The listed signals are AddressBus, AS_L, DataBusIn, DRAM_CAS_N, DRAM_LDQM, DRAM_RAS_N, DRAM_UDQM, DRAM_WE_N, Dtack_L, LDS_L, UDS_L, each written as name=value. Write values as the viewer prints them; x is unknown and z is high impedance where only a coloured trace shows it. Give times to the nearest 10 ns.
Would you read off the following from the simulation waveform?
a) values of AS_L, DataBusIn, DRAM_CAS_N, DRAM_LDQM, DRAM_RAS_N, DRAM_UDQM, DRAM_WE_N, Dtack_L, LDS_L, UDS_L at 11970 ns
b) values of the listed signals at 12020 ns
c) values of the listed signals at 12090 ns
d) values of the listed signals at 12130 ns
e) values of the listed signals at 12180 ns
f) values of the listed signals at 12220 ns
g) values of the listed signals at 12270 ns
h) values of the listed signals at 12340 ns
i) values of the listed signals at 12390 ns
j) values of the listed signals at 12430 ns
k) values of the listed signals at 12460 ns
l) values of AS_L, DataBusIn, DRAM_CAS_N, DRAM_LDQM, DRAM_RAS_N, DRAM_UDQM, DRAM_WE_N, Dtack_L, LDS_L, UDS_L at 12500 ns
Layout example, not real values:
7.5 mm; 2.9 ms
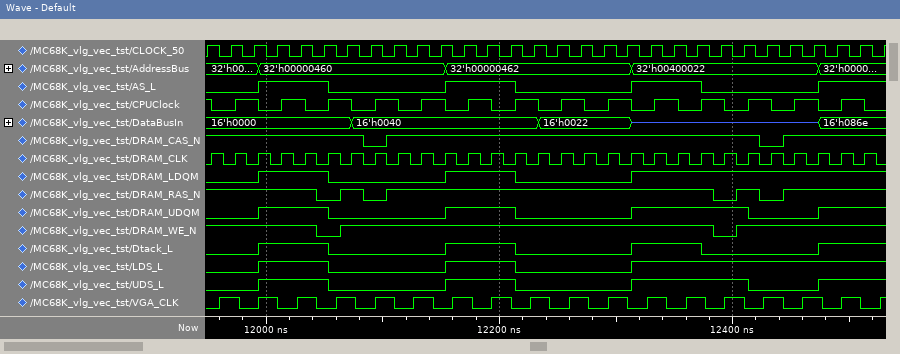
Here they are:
AS_L=0, DataBusIn=16'h0000, DRAM_CAS_N=1, DRAM_LDQM=0, DRAM_RAS_N=1, DRAM_UDQM=0, DRAM_WE_N=1, Dtack_L=0, LDS_L=0, UDS_L=0; AddressBus=32'h00000460, AS_L=1, DataBusIn=16'h0000, DRAM_CAS_N=1, DRAM_LDQM=1, DRAM_RAS_N=1, DRAM_UDQM=1, DRAM_WE_N=1, Dtack_L=1, LDS_L=1, UDS_L=1; AddressBus=32'h00000460, AS_L=0, DataBusIn=16'h0040, DRAM_CAS_N=0, DRAM_LDQM=0, DRAM_RAS_N=0, DRAM_UDQM=0, DRAM_WE_N=1, Dtack_L=0, LDS_L=0, UDS_L=0; AddressBus=32'h00000460, AS_L=0, DataBusIn=16'h0040, DRAM_CAS_N=1, DRAM_LDQM=0, DRAM_RAS_N=1, DRAM_UDQM=0, DRAM_WE_N=1, Dtack_L=0, LDS_L=0, UDS_L=0; AddressBus=32'h00000462, AS_L=1, DataBusIn=16'h0040, DRAM_CAS_N=1, DRAM_LDQM=1, DRAM_RAS_N=1, DRAM_UDQM=1, DRAM_WE_N=1, Dtack_L=1, LDS_L=1, UDS_L=1; AddressBus=32'h00000462, AS_L=0, DataBusIn=16'h0040, DRAM_CAS_N=1, DRAM_LDQM=0, DRAM_RAS_N=1, DRAM_UDQM=0, DRAM_WE_N=1, Dtack_L=0, LDS_L=0, UDS_L=0; AddressBus=32'h00000462, AS_L=0, DataBusIn=16'h0022, DRAM_CAS_N=1, DRAM_LDQM=0, DRAM_RAS_N=1, DRAM_UDQM=0, DRAM_WE_N=1, Dtack_L=0, LDS_L=0, UDS_L=0; AddressBus=32'h00400022, AS_L=1, DataBusIn=z, DRAM_CAS_N=1, DRAM_LDQM=1, DRAM_RAS_N=1, DRAM_UDQM=1, DRAM_WE_N=1, Dtack_L=1, LDS_L=1, UDS_L=1; AddressBus=32'h00400022, AS_L=0, DataBusIn=z, DRAM_CAS_N=1, DRAM_LDQM=1, DRAM_RAS_N=0, DRAM_UDQM=1, DRAM_WE_N=0, Dtack_L=0, LDS_L=1, UDS_L=1; AddressBus=32'h00400022, AS_L=0, DataBusIn=z, DRAM_CAS_N=0, DRAM_LDQM=1, DRAM_RAS_N=0, DRAM_UDQM=0, DRAM_WE_N=1, Dtack_L=0, LDS_L=1, UDS_L=0; AddressBus=32'h00400022, AS_L=0, DataBusIn=z, DRAM_CAS_N=1, DRAM_LDQM=1, DRAM_RAS_N=1, DRAM_UDQM=0, DRAM_WE_N=1, Dtack_L=0, LDS_L=1, UDS_L=0; AS_L=1, DataBusIn=16'h086e, DRAM_CAS_N=1, DRAM_LDQM=1, DRAM_RAS_N=1, DRAM_UDQM=1, DRAM_WE_N=1, Dtack_L=1, LDS_L=1, UDS_L=1
